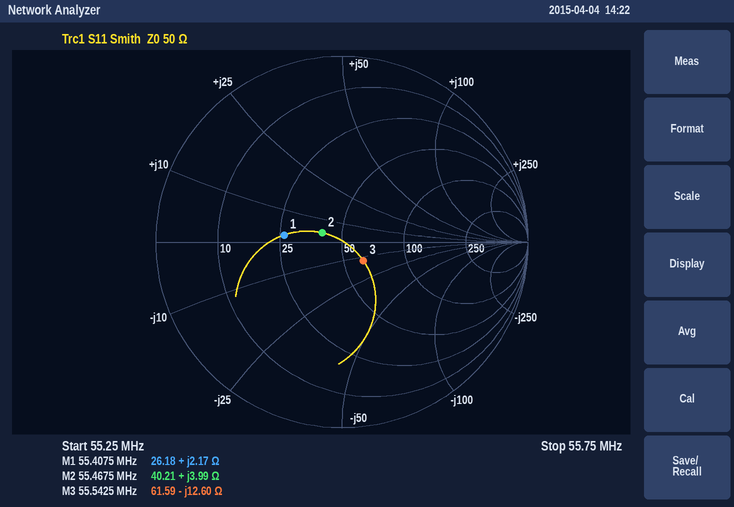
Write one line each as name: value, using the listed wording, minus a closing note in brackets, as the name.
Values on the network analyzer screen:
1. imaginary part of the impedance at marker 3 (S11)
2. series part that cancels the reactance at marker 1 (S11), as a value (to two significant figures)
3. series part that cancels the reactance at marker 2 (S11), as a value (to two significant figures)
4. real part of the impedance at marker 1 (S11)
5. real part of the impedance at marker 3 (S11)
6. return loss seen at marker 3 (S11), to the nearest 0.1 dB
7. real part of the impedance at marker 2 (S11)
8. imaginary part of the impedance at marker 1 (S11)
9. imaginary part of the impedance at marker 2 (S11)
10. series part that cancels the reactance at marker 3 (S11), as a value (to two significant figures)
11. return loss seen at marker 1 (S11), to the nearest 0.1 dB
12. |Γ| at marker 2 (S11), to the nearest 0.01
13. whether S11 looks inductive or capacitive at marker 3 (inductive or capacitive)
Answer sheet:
imaginary part of the impedance at marker 3: -12.60 Ω
series part that cancels the reactance at marker 1 (S11), as a value: 1.3 nF
series part that cancels the reactance at marker 2 (S11), as a value: 720 pF
real part of the impedance at marker 1: 26.18 Ω
real part of the impedance at marker 3: 61.59 Ω
return loss seen at marker 3 (S11), to the nearest 0.1 dB: 16.3 dB
real part of the impedance at marker 2: 40.21 Ω
imaginary part of the impedance at marker 1: +2.17 Ω
imaginary part of the impedance at marker 2: +3.99 Ω
series part that cancels the reactance at marker 3 (S11), as a value: 36 nH
return loss seen at marker 1 (S11), to the nearest 0.1 dB: 10.1 dB
|Γ| at marker 2 (S11), to the nearest 0.01: 0.12
whether S11 looks inductive or capacitive at marker 3: capacitive
